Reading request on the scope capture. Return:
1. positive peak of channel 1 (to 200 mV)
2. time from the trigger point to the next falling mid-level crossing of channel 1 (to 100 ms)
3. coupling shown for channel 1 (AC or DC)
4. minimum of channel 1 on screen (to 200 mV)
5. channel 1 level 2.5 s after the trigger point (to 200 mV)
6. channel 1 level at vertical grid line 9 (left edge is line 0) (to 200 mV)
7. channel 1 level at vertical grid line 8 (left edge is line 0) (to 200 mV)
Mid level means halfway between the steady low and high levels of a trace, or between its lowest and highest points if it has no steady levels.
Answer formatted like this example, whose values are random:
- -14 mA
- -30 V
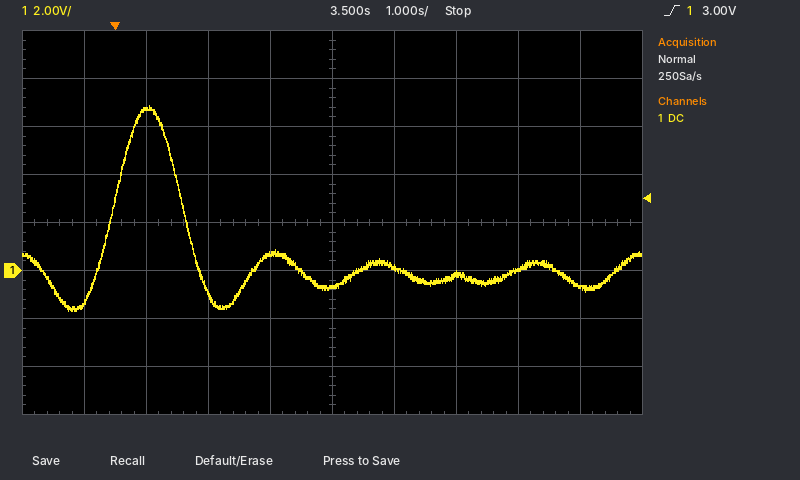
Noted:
- 6.8 V
- 1.1 s
- DC
- -1.6 V
- 800 mV
- -600 mV
- 0.0 V
